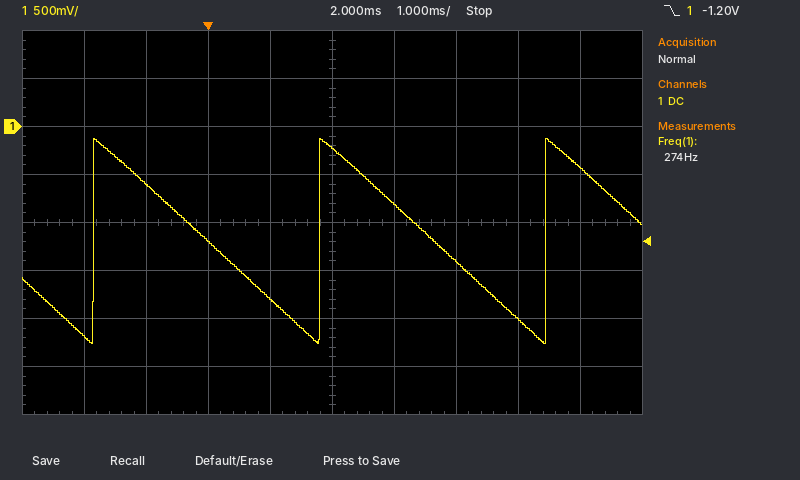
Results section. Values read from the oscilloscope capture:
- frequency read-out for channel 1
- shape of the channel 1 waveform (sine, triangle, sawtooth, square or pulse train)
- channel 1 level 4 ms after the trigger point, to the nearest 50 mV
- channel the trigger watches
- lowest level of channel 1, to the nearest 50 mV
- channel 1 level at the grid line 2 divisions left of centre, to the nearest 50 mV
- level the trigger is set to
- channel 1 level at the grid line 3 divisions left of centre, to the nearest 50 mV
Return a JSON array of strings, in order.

["274 Hz", "sawtooth", "-1.40 V", "channel 1", "-2.25 V", "-1.20 V", "-1.20 V", "-600 mV"]
